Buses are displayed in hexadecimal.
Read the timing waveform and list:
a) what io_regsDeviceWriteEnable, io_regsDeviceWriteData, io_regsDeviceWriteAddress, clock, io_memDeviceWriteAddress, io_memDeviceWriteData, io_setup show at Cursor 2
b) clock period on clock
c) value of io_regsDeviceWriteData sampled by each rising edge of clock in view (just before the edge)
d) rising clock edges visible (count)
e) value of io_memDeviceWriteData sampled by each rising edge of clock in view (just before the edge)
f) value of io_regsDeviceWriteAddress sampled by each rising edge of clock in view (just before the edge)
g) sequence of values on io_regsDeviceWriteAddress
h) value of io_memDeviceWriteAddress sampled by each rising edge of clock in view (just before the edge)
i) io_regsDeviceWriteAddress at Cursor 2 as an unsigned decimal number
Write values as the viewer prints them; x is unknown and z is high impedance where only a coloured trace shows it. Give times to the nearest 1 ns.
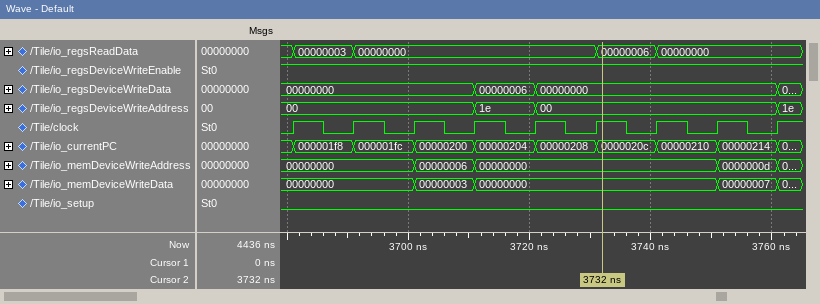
io_regsDeviceWriteEnable=1, io_regsDeviceWriteData=00000000, io_regsDeviceWriteAddress=00, clock=1, io_memDeviceWriteAddress=00000000, io_memDeviceWriteData=00000000, io_setup=0
10 ns
00000000, 00000000, 00000000, 00000000, 00000006, 00000000, 00000000, 00000000, 00000000
9
00000000, 00000000, 00000000, 00000003, 00000000, 00000000, 00000000, 00000000, 00000007
00, 00, 00, 00, 1e, 00, 00, 00, 00
00, 1e, 00, 1e
00000000, 00000000, 00000000, 00000006, 00000000, 00000000, 00000000, 00000000, 0000000d
0
